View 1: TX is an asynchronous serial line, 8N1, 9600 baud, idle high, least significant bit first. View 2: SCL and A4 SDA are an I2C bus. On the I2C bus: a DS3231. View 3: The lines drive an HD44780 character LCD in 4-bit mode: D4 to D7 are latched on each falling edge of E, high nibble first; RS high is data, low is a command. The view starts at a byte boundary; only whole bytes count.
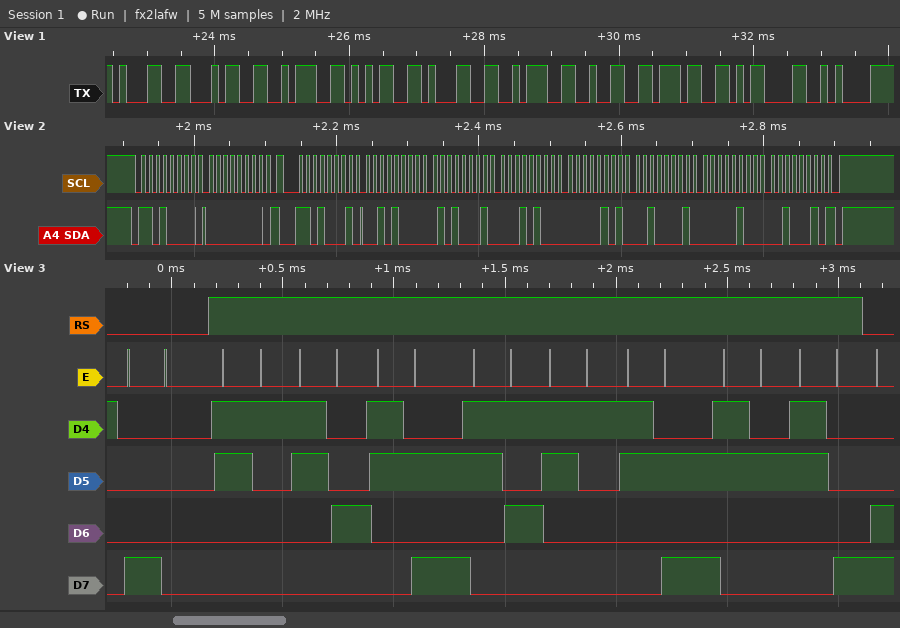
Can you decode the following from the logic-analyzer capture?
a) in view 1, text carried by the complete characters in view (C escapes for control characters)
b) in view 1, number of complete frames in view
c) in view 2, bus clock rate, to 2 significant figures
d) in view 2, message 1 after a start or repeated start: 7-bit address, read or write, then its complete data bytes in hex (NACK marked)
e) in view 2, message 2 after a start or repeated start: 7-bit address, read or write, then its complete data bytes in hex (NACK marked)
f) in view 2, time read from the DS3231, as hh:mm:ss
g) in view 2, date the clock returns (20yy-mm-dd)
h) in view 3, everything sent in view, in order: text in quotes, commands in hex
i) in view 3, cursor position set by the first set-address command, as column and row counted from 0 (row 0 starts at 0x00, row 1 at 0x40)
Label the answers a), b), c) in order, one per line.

a) "14:51:27\r\n"
b) 10
c) 100 kHz
d) 0x68 write: 00
e) 0x68 read: 28 51 14 05 21 04 22 NACK
f) 14:51:28
g) 2022-04-21
h) 0x80 "14:51:28"
i) column 0, row 0
